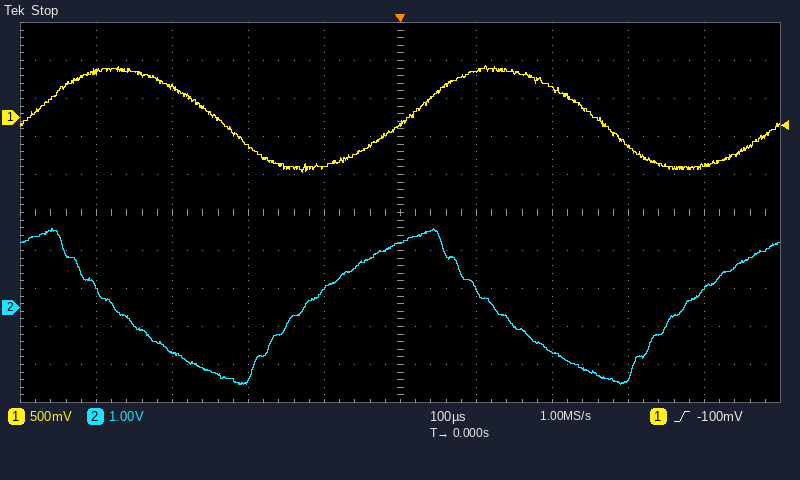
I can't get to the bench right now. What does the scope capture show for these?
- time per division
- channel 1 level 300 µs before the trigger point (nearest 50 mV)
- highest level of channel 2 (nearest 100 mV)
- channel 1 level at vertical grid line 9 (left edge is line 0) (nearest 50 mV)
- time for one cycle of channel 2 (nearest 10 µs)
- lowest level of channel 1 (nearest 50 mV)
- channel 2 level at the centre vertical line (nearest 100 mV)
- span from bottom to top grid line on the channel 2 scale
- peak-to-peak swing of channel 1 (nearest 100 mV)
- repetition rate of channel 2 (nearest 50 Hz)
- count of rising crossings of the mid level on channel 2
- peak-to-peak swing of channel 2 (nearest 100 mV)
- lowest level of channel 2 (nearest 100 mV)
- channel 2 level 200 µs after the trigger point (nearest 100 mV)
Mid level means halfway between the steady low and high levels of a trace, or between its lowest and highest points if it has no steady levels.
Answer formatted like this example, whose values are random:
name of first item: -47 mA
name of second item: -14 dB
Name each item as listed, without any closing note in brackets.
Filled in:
time per division: 100 µs
channel 1 level 300 µs before the trigger point: 400 mV
highest level of channel 2: 2.1 V
channel 1 level at vertical grid line 9 (left edge is line 0): -650 mV
time for one cycle of channel 2: 500 µs
lowest level of channel 1: -700 mV
channel 2 level at the centre vertical line: 1.7 V
span from bottom to top grid line on the channel 2 scale: 10 V
peak-to-peak swing of channel 1: 1.40 V
repetition rate of channel 2: 2.00 kHz
count of rising crossings of the mid level on channel 2: 2
peak-to-peak swing of channel 2: 4.1 V
lowest level of channel 2: -2.0 V
channel 2 level 200 µs after the trigger point: -1.2 V
